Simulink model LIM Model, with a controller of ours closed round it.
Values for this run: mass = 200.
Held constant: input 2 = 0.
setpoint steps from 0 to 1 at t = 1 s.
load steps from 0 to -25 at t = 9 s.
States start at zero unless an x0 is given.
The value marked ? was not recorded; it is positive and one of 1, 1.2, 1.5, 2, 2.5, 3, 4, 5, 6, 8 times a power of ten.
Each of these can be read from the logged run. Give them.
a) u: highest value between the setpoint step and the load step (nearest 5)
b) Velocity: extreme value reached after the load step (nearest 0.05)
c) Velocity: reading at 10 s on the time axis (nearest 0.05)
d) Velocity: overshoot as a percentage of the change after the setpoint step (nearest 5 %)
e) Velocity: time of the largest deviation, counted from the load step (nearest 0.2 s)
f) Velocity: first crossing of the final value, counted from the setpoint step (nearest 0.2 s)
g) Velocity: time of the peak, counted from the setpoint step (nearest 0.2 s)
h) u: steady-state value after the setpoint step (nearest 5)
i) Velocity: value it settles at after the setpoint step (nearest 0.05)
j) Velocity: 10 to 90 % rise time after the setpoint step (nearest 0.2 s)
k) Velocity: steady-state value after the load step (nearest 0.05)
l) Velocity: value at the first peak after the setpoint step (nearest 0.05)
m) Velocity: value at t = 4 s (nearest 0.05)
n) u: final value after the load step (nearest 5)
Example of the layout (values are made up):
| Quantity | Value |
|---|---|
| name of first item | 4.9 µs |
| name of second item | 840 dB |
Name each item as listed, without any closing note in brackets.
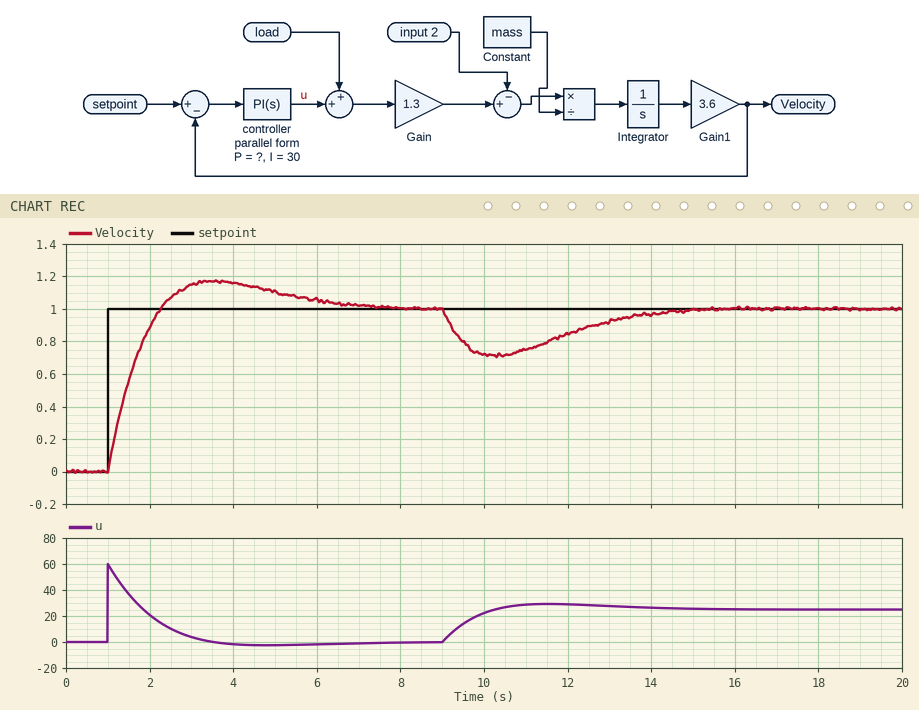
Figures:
| Quantity | Value |
|---|---|
| u: highest value between the setpoint step and the load step | 60 |
| Velocity: extreme value reached after the load step | 0.70 |
| Velocity: reading at 10 s on the time axis | 0.70 |
| Velocity: overshoot as a percentage of the change after the setpoint step | 15 % |
| Velocity: time of the largest deviation, counted from the load step | 1.2 s |
| Velocity: first crossing of the final value, counted from the setpoint step | 1.2 s |
| Velocity: time of the peak, counted from the setpoint step | 2.6 s |
| u: steady-state value after the setpoint step | 0 |
| Velocity: value it settles at after the setpoint step | 1.00 |
| Velocity: 10 to 90 % rise time after the setpoint step | 1.0 s |
| Velocity: steady-state value after the load step | 1.00 |
| Velocity: value at the first peak after the setpoint step | 1.15 |
| Velocity: value at t = 4 s | 1.15 |
| u: final value after the load step | 25 |
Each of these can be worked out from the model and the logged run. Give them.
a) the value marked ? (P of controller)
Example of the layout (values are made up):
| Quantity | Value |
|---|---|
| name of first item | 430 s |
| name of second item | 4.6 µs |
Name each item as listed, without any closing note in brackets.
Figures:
| Quantity | Value |
|---|---|
| the value marked ? | 60 |
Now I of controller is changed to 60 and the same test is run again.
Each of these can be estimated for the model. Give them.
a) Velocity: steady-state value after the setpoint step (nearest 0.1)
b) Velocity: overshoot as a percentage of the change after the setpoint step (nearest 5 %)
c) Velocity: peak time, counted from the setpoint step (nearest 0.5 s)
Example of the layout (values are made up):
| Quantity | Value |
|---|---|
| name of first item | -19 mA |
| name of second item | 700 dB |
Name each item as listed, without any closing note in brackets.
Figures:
| Quantity | Value |
|---|---|
| Velocity: steady-state value after the setpoint step | 1.0 |
| Velocity: overshoot as a percentage of the change after the setpoint step | 25 % |
| Velocity: peak time, counted from the setpoint step | 2.0 s |
